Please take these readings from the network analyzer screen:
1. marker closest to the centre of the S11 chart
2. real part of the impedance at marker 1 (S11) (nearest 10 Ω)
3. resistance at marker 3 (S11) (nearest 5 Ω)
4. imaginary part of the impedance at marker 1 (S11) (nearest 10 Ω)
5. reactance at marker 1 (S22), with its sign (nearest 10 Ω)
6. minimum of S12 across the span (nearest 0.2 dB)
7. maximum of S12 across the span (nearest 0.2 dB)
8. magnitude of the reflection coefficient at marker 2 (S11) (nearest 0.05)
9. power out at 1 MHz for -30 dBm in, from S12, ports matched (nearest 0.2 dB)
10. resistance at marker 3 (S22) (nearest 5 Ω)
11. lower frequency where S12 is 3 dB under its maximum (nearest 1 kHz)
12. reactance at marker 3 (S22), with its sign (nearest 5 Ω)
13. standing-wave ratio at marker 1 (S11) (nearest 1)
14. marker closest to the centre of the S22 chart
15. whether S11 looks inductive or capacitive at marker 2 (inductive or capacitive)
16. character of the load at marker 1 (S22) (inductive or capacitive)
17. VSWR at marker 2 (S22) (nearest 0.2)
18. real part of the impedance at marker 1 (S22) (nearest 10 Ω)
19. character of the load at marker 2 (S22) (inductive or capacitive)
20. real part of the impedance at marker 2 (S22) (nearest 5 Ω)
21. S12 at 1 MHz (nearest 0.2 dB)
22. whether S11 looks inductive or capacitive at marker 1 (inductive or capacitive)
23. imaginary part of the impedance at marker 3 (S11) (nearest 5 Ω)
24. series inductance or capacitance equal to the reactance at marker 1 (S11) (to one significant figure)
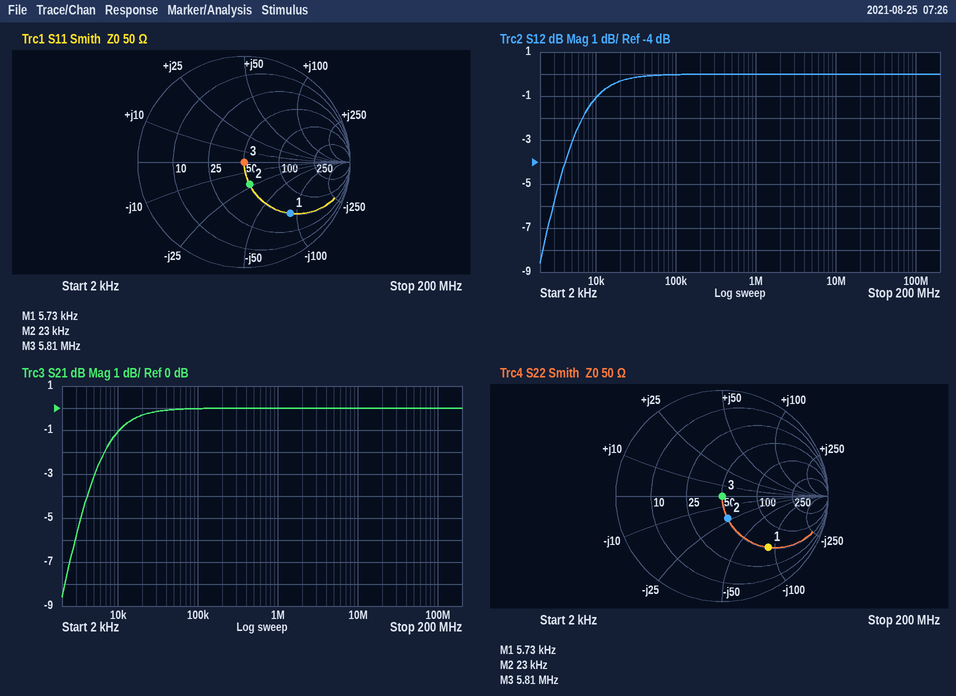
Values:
marker 3
50 Ω
50 Ω
-90 Ω
-90 Ω
-8.6 dB
0.0 dB
0.20
-30.0 dBm
50 Ω
5 kHz
0 Ω
5
marker 3
capacitive
capacitive
1.6
50 Ω
capacitive
50 Ω
0.0 dB
capacitive
0 Ω
300 nF
